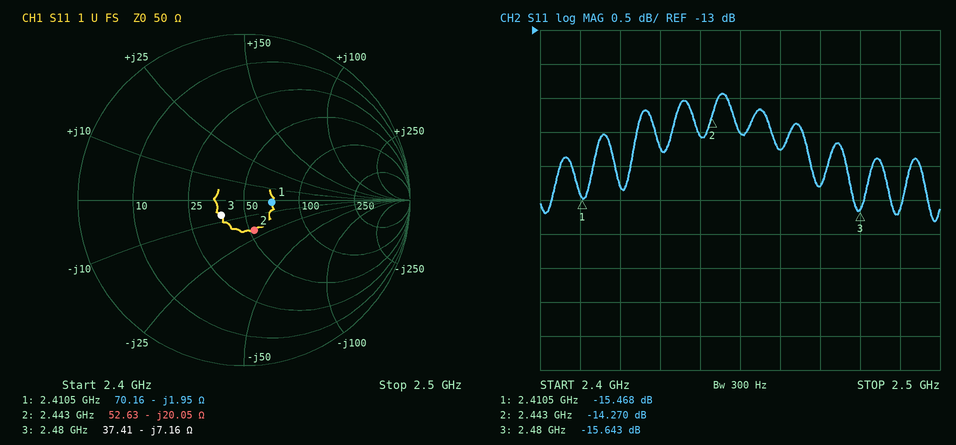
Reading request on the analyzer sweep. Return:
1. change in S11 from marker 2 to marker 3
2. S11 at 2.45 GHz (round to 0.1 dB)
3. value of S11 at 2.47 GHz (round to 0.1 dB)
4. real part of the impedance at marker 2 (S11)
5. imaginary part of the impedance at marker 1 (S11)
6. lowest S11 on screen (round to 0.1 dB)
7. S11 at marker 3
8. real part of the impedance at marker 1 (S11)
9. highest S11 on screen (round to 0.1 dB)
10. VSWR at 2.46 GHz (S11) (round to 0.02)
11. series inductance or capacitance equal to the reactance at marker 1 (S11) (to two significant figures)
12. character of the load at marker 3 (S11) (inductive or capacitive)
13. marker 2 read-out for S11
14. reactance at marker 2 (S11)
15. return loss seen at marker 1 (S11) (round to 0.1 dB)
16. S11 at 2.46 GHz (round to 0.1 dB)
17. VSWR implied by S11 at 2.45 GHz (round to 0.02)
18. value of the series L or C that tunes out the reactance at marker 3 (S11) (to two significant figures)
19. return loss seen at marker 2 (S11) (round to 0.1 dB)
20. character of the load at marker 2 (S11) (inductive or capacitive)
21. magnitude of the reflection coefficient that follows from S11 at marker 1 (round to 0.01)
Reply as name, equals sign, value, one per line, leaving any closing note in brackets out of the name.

change in S11 from marker 2 to marker 3 = -1.373 dB
S11 at 2.45 GHz = -14.5 dB
value of S11 at 2.47 GHz = -15.3 dB
real part of the impedance at marker 2 = 52.63 Ω
imaginary part of the impedance at marker 1 = -1.95 Ω
lowest S11 on screen = -15.8 dB
S11 at marker 3 = -15.643 dB
real part of the impedance at marker 1 = 70.16 Ω
highest S11 on screen = -13.9 dB
VSWR at 2.46 GHz (S11) = 1.44
series inductance or capacitance equal to the reactance at marker 1 (S11) = 34 pF
character of the load at marker 3 (S11) = capacitive
marker 2 read-out for S11 = -14.270 dB
reactance at marker 2 = -20.05 Ω
return loss seen at marker 1 (S11) = 15.5 dB
S11 at 2.46 GHz = -14.8 dB
VSWR implied by S11 at 2.45 GHz = 1.46
value of the series L or C that tunes out the reactance at marker 3 (S11) = 460 pH
return loss seen at marker 2 (S11) = 14.3 dB
character of the load at marker 2 (S11) = capacitive
magnitude of the reflection coefficient that follows from S11 at marker 1 = 0.17
